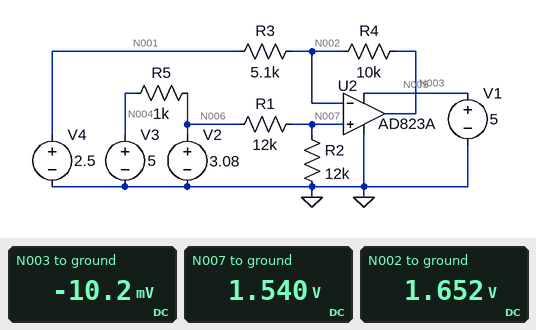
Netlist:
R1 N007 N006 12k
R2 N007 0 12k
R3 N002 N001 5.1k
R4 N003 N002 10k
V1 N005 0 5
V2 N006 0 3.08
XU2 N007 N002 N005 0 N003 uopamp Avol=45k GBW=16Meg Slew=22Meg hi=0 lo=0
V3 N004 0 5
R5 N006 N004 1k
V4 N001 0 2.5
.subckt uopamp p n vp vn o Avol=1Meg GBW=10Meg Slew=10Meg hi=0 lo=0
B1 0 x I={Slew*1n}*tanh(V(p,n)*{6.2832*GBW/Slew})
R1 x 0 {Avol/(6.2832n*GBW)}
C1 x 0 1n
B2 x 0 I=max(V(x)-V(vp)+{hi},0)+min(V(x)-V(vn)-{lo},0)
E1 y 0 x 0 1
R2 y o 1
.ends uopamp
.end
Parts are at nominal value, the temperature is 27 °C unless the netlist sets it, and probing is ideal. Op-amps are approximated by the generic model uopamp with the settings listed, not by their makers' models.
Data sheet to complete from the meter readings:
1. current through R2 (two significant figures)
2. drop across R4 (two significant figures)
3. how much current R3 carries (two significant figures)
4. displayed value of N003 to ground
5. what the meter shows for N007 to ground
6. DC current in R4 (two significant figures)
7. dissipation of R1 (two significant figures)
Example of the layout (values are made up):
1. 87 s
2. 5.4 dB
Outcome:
1. 130 µA
2. 1.7 V
3. 170 µA
4. -10.2 mV
5. 1.540 V
6. 170 µA
7. 200 µW
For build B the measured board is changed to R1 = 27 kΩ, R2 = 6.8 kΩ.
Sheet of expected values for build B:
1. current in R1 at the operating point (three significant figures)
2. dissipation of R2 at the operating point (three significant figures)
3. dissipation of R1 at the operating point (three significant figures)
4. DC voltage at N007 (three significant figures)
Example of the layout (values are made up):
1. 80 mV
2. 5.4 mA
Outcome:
1. 91.1 µA
2. 56.5 µW
3. 224 µW
4. 620 mV
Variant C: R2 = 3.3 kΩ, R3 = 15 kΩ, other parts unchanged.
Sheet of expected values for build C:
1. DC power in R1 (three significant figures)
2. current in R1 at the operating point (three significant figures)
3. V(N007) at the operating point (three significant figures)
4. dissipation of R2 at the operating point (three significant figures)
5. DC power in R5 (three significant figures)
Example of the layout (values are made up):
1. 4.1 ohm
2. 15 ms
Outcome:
1. 486 µW
2. 201 µA
3. 664 mV
4. 134 µW
5. 3.69 mW
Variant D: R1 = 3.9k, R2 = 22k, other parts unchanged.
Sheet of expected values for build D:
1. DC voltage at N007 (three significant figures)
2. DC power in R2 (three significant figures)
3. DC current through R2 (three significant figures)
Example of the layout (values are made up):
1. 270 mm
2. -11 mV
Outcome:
1. 2.62 V
2. 311 µW
3. 119 µA
